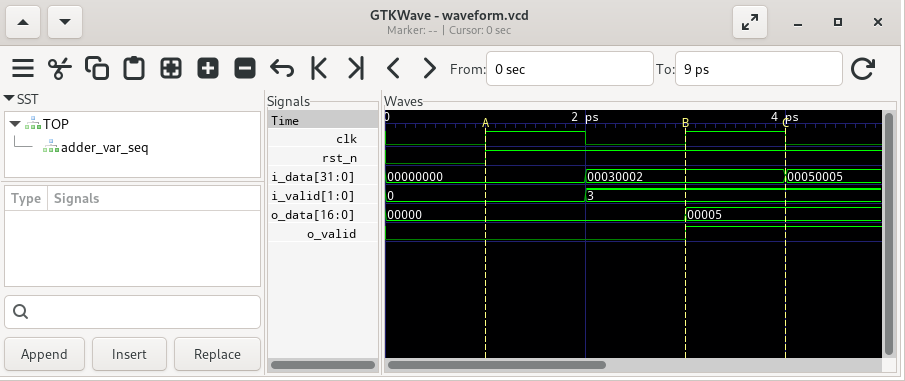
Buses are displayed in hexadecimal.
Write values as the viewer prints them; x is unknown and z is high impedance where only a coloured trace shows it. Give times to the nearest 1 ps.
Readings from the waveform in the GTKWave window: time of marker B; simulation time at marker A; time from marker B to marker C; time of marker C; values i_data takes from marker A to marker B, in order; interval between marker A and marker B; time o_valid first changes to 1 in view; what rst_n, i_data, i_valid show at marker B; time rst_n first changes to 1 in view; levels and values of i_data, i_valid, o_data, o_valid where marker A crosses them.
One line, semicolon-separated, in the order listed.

3 ps; 1 ps; 1 ps; 4 ps; 00000000, 00030002; 2 ps; 3 ps; rst_n=1, i_data=00030002, i_valid=3; 1 ps; i_data=00000000, i_valid=0, o_data=00000, o_valid=0
